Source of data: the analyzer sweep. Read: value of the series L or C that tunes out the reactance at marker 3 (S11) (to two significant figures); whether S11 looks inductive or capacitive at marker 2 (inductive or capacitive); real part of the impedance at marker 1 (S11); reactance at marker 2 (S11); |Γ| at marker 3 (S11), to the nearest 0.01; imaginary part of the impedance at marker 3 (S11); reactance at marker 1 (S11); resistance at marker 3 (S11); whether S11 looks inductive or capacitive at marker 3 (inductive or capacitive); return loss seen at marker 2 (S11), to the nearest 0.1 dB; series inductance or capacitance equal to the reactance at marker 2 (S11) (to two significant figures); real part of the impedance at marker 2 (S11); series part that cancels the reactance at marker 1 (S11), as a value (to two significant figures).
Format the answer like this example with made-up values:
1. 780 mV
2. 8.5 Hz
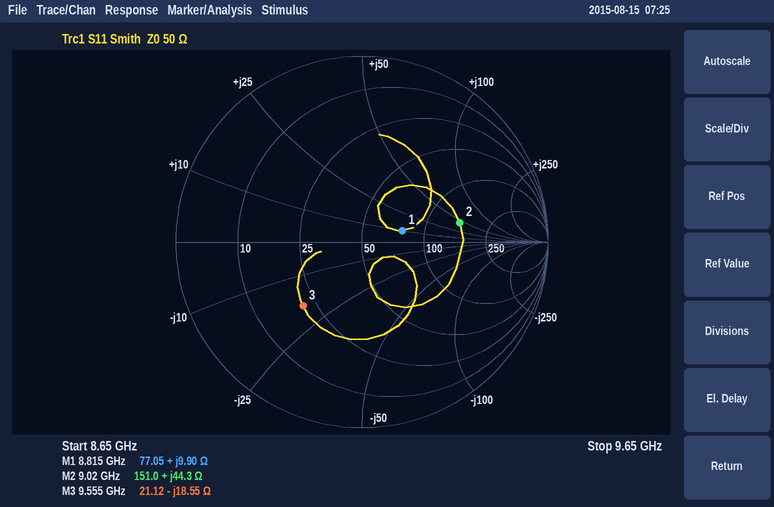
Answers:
1. 310 pH
2. inductive
3. 77.05 Ω
4. +44.3 Ω
5. 0.47
6. -18.55 Ω
7. +9.90 Ω
8. 21.12 Ω
9. capacitive
10. 5.4 dB
11. 780 pH
12. 151.0 Ω
13. 1.8 pF
